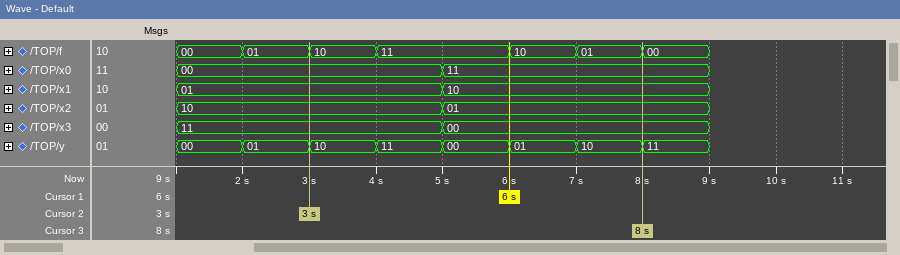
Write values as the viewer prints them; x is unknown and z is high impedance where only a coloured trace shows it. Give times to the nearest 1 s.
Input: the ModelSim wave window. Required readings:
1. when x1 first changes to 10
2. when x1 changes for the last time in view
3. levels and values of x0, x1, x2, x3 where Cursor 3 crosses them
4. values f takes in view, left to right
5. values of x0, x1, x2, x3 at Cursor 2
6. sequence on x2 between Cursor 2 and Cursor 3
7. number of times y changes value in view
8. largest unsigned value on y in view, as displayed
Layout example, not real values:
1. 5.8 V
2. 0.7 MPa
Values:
1. 5 s
2. 5 s
3. x0=11, x1=10, x2=01, x3=00
4. 00, 01, 10, 11, 10, 01, 00
5. x0=00, x1=01, x2=10, x3=11
6. 10, 01
7. 7
8. 11
